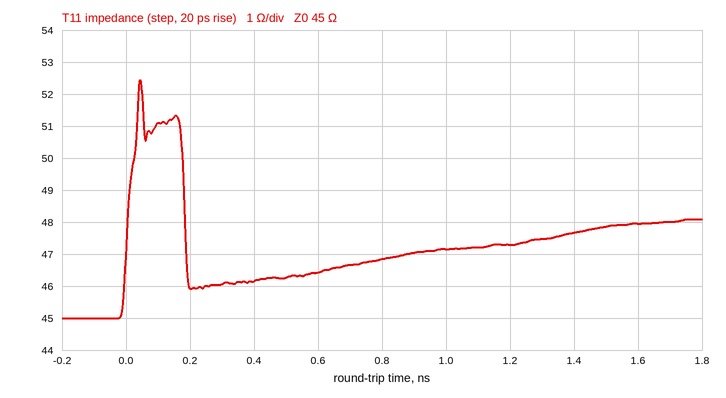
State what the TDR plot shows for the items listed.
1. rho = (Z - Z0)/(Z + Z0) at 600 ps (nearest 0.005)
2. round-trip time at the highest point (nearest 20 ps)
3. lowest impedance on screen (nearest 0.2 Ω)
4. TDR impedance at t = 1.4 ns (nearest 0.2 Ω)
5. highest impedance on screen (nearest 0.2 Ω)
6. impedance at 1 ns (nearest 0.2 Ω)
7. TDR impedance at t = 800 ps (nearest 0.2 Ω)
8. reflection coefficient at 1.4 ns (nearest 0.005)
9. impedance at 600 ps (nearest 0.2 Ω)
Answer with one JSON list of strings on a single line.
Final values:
["+0.015", "40 ps", "45.0 Ω", "47.6 Ω", "52.4 Ω", "47.2 Ω", "46.8 Ω", "+0.030", "46.4 Ω"]
